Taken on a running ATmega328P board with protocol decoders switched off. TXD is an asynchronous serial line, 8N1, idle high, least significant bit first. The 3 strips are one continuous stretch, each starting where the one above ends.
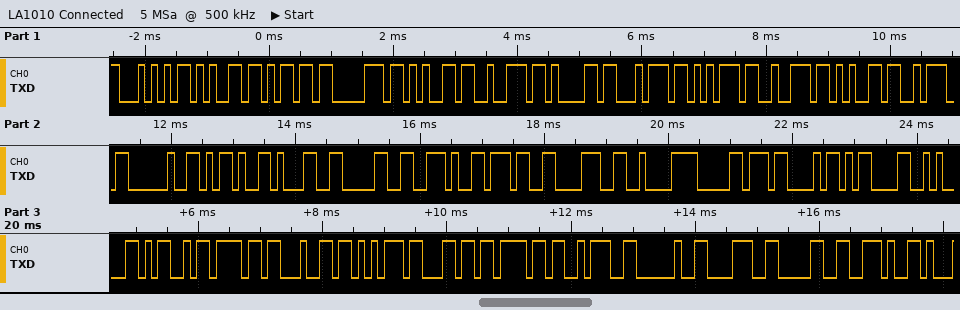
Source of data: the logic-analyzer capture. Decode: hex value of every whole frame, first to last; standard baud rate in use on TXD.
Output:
54 65 6D 70 65 72 61 74 75 72 65 3A 20 2D 31 30 2E 37 38 C2 B0 43 0D 0A 4D 6F 64 75 6C 6F 3A 20 38 30 2E
9600 baud
